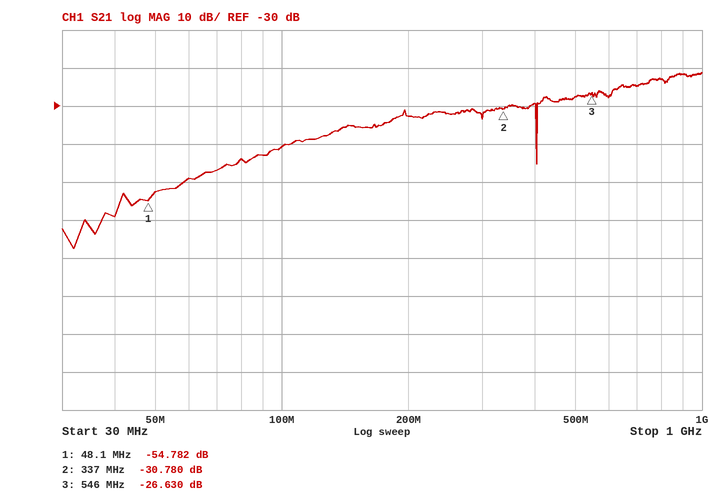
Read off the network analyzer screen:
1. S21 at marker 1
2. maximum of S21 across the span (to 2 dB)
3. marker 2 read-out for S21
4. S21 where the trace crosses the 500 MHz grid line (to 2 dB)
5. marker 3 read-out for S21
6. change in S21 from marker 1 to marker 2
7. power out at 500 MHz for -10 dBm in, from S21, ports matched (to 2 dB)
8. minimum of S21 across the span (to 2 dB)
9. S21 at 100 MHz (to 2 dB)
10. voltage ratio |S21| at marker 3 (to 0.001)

-54.782 dB
-22 dB
-30.780 dB
-28 dB
-26.630 dB
24.002 dB
-38 dBm
-68 dB
-40 dB
0.047
